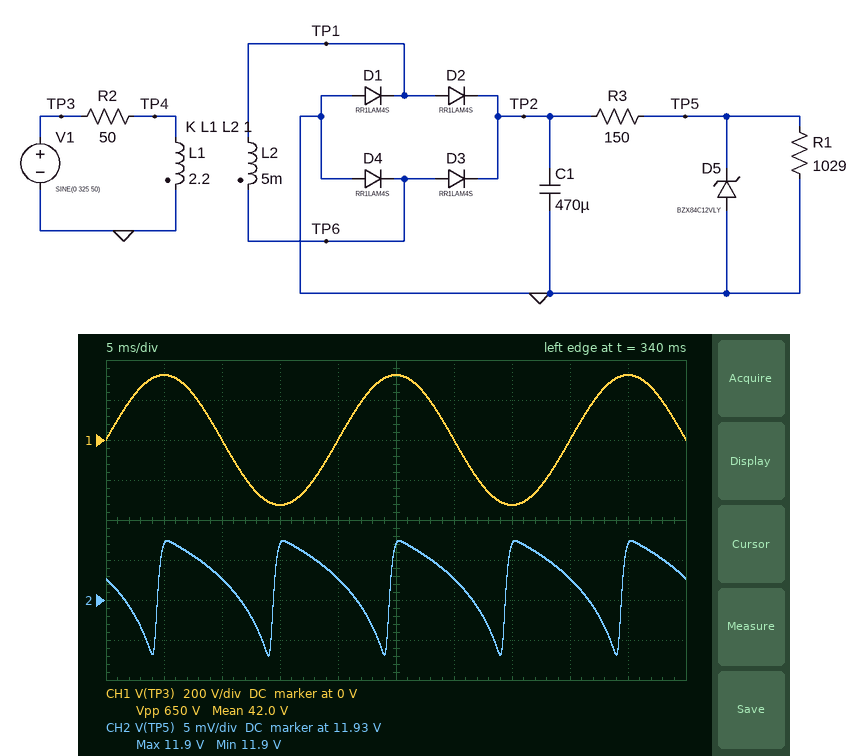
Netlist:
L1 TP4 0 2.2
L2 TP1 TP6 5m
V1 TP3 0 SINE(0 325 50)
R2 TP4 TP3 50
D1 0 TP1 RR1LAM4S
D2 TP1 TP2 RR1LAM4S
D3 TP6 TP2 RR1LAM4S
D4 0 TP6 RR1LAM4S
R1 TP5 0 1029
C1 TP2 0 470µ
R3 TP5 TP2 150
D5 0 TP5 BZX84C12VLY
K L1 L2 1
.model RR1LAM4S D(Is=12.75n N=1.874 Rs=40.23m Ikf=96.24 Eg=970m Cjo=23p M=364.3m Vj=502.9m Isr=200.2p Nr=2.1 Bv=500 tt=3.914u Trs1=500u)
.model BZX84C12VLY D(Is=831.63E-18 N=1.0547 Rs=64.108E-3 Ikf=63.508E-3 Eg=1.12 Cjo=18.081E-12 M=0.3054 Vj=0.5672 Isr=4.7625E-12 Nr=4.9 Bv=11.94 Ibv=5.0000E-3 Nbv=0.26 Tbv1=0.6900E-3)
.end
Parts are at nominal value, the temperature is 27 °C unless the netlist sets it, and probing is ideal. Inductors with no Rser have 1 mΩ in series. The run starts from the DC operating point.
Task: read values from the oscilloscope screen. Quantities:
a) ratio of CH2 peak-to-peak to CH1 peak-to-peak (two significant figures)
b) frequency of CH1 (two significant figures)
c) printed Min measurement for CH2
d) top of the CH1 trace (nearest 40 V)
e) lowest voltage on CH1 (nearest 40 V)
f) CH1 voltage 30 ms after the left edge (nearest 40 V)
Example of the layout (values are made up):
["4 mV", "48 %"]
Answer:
["0.000022", "50 Hz", "11.9 V", "320 V", "-320 V", "0 V"]
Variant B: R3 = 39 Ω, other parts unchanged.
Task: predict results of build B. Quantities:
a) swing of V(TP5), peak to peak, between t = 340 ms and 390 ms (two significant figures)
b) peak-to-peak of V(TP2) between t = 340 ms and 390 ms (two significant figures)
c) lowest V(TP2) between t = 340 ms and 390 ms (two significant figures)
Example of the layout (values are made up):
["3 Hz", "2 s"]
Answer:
["5.5 mV", "700 mV", "13 V"]
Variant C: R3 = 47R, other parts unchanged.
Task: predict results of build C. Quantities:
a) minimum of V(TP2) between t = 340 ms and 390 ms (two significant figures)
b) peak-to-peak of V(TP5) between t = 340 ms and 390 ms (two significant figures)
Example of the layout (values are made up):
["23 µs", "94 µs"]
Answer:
["13 V", "4.7 mV"]
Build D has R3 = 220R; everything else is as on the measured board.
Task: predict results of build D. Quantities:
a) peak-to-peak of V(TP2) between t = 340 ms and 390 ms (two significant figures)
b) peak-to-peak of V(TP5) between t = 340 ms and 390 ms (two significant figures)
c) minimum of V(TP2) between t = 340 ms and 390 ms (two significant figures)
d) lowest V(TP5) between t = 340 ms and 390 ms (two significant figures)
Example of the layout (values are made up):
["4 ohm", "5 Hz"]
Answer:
["200 mV", "170 mV", "14 V", "11 V"]
